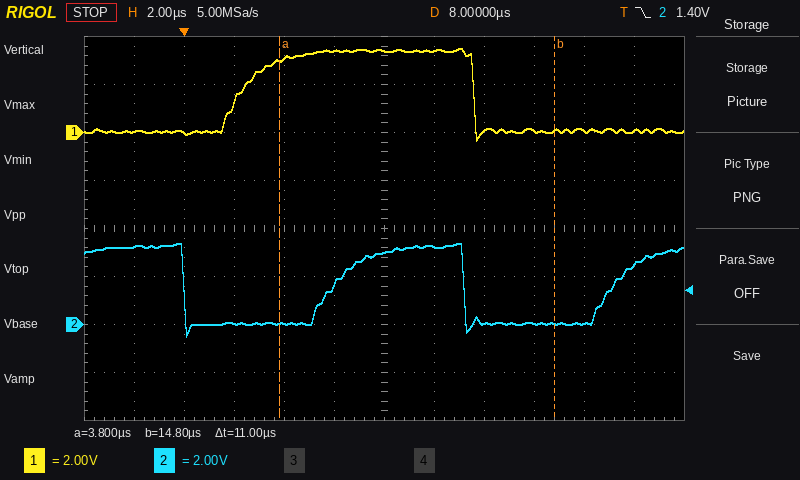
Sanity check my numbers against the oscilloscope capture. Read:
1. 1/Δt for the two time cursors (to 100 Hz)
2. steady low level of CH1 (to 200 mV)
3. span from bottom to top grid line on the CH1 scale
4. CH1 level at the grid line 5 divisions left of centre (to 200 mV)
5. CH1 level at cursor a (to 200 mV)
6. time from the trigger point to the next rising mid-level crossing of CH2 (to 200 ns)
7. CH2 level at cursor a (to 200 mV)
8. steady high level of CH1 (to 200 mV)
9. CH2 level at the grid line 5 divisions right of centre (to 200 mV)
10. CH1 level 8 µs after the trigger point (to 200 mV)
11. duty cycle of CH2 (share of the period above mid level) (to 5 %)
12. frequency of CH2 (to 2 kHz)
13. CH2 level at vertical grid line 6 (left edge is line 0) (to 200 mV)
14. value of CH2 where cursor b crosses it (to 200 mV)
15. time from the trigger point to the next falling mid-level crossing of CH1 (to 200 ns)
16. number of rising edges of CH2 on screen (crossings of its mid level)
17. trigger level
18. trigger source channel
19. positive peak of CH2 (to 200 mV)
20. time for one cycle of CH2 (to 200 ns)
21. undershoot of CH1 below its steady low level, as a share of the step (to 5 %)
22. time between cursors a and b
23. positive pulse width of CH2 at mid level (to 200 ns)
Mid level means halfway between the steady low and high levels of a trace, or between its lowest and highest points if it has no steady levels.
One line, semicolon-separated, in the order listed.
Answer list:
90.9 kHz; 0.0 V; 16 V; 0.0 V; 3.0 V; 6.0 µs; 0.0 V; 3.4 V; 2.4 V; 3.4 V; 45 %; 90 kHz; 3.0 V; 0.0 V; 11.6 µs; 2; 1.40 V; CH2; 3.4 V; 11.2 µs; 10 %; 11 µs; 5.2 µs
